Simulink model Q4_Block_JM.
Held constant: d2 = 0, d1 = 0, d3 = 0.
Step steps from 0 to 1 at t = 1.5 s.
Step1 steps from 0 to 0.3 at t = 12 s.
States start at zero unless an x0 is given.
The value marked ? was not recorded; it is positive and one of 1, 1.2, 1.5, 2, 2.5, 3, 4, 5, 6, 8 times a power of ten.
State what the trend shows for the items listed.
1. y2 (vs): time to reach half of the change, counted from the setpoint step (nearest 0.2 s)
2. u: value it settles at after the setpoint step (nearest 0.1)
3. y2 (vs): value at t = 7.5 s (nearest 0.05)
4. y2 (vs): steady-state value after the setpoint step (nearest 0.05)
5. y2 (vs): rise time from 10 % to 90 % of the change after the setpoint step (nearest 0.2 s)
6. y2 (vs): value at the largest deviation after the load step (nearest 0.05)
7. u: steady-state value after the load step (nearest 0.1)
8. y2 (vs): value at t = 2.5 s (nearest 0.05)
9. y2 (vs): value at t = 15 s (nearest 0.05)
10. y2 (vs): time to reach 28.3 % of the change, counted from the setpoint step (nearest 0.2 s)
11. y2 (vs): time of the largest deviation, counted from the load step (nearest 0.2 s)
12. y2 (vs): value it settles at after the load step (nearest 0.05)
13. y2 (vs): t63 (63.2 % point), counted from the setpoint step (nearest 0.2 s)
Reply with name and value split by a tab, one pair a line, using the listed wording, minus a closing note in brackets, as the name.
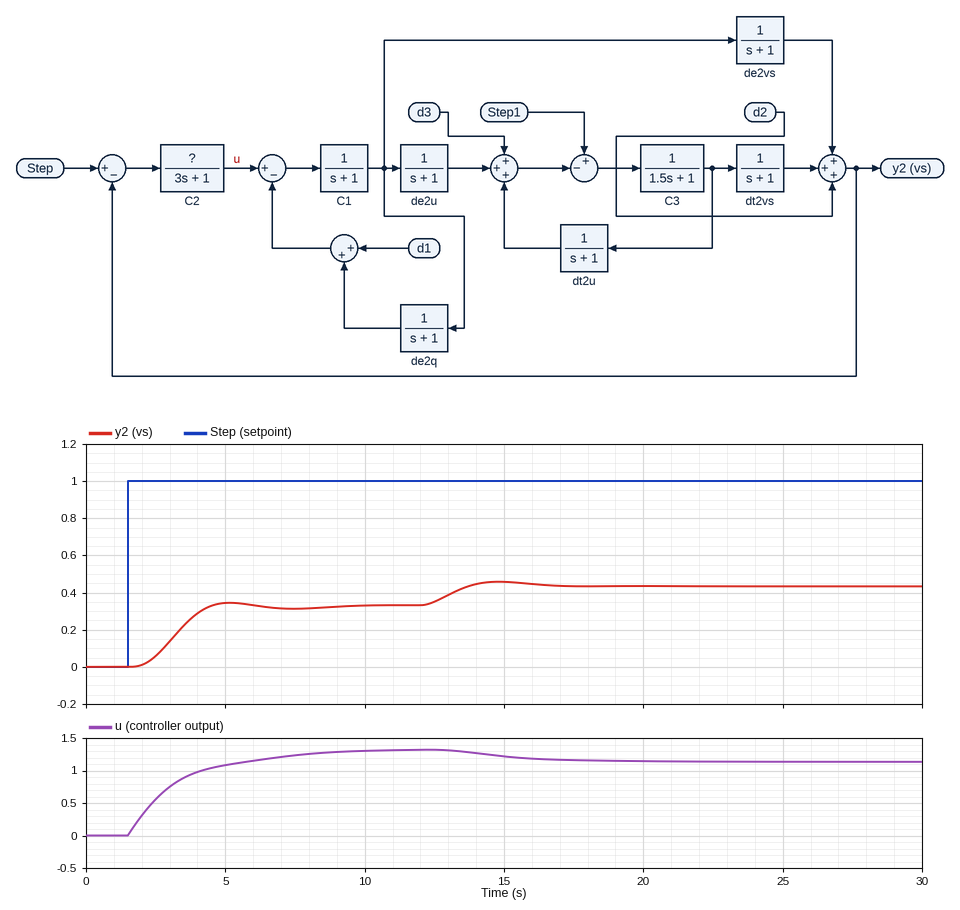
y2 (vs): time to reach half of the change, counted from the setpoint step	1.6 s
u: value it settles at after the setpoint step	1.3
y2 (vs): value at t = 7.5 s	0.30
y2 (vs): steady-state value after the setpoint step	0.35
y2 (vs): rise time from 10 % to 90 % of the change after the setpoint step	1.8 s
y2 (vs): value at the largest deviation after the load step	0.45
u: steady-state value after the load step	1.1
y2 (vs): value at t = 2.5 s	0.05
y2 (vs): value at t = 15 s	0.45
y2 (vs): time to reach 28.3 % of the change, counted from the setpoint step	1.2 s
y2 (vs): time of the largest deviation, counted from the load step	2.8 s
y2 (vs): value it settles at after the load step	0.45
y2 (vs): t63 (63.2 % point), counted from the setpoint step	2.0 s
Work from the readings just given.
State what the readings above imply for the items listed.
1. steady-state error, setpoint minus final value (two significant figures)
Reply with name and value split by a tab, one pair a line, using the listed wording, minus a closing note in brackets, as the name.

steady-state error, setpoint minus final value	0.65
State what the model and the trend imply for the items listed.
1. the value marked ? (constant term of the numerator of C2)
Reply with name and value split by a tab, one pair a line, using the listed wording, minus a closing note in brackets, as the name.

the value marked ?	2
